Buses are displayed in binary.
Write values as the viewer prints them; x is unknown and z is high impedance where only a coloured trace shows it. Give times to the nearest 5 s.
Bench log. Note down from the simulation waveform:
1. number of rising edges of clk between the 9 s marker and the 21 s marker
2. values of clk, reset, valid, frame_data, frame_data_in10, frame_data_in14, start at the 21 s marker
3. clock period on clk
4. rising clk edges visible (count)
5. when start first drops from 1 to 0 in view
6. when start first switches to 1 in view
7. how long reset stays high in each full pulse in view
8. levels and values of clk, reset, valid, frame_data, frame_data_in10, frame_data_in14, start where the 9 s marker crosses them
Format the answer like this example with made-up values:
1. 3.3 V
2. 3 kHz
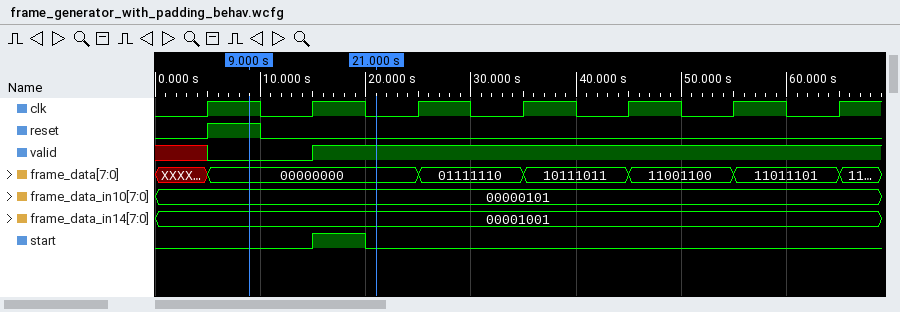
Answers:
1. 1
2. clk=0, reset=0, valid=1, frame_data=00000000, frame_data_in10=00000101, frame_data_in14=00001001, start=0
3. 10 s
4. 7
5. 20 s
6. 15 s
7. 5 s
8. clk=1, reset=1, valid=0, frame_data=00000000, frame_data_in10=00000101, frame_data_in14=00001001, start=0
